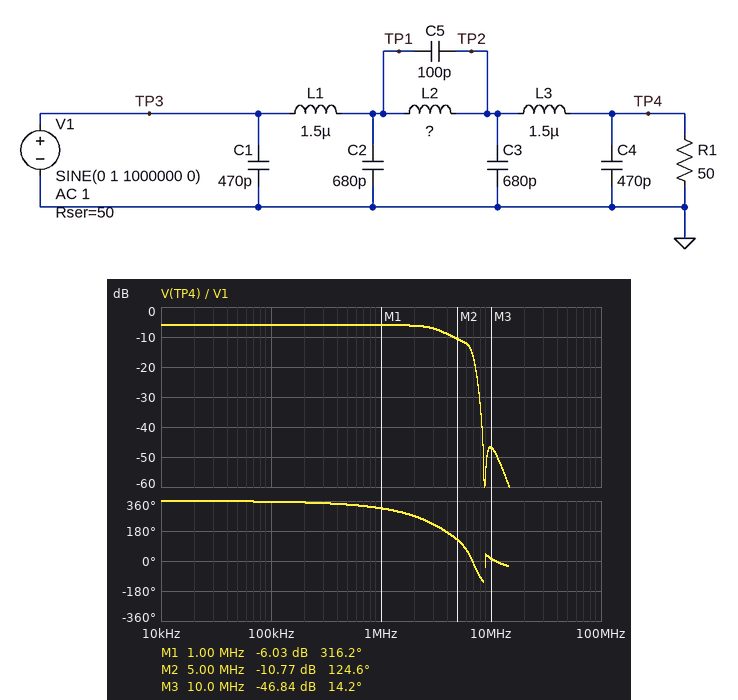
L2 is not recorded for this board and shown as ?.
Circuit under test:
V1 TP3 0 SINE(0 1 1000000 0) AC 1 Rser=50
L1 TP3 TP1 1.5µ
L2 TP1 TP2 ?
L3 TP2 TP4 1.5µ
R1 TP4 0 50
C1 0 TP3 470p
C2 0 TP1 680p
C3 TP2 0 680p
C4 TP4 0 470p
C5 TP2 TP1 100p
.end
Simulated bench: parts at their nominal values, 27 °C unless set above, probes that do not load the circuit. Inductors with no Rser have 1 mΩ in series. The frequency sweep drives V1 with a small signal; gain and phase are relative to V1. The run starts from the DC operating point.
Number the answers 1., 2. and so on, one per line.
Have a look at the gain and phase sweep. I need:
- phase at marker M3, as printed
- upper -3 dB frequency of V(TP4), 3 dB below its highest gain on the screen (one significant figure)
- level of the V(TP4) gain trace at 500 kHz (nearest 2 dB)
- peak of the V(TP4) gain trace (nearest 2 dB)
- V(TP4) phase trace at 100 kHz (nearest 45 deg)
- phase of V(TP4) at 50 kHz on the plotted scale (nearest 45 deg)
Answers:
1. 14.2 deg
2. 4 MHz
3. -6 dB
4. -6 dB
5. 360 deg
6. 360 deg
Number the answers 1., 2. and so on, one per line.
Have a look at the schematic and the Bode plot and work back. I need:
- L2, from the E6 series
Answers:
1. 3.3 µH
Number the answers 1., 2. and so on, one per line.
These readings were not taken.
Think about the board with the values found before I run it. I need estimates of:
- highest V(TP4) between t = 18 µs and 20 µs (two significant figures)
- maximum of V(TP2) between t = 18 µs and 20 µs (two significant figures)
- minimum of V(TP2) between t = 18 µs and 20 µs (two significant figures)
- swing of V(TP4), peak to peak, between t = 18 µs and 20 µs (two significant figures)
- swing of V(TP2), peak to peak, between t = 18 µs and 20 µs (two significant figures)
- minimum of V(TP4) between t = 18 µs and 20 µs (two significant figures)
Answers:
1. 500 mV
2. 490 mV
3. -490 mV
4. 1.0 V
5. 990 mV
6. -500 mV
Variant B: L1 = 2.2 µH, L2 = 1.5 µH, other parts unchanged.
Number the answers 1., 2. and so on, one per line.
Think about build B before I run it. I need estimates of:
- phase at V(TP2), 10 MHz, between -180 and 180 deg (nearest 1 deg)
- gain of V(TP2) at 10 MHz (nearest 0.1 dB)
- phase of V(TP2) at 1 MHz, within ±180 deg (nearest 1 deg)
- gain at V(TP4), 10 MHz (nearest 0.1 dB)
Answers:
1. -39 deg
2. -30.9 dB
3. -29 deg
4. -39.2 dB
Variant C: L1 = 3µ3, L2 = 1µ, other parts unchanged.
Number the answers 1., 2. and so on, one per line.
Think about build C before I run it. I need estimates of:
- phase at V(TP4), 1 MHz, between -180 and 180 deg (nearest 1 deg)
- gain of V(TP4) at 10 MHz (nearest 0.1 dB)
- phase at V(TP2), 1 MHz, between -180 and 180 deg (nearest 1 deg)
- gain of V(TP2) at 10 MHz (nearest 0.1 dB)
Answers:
1. -42 deg
2. -32.2 dB
3. -31 deg
4. -23.9 dB
